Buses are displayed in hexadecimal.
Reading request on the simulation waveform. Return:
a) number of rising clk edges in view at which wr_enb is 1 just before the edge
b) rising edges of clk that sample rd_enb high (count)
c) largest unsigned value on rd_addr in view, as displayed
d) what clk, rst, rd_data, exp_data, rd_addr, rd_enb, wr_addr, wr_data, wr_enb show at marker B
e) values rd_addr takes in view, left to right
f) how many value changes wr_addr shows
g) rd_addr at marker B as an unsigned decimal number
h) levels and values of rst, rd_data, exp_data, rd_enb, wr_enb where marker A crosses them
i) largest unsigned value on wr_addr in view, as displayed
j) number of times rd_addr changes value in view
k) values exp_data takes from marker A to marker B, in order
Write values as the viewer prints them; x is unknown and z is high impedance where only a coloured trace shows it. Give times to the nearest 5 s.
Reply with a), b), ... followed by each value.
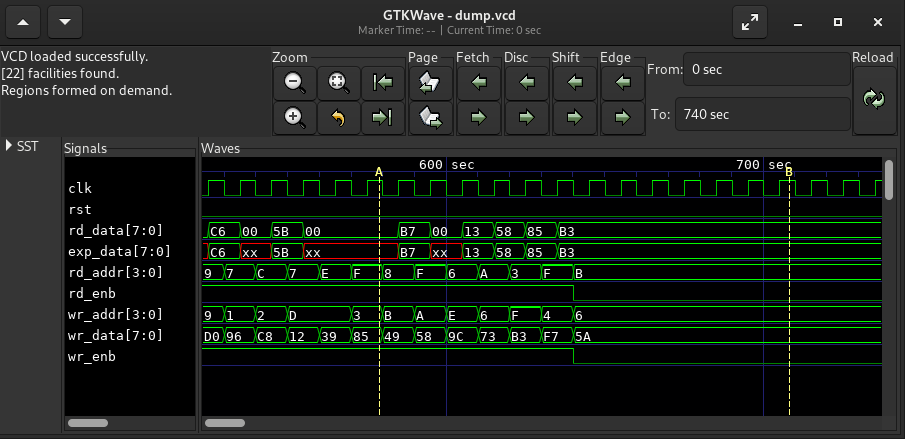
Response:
a) 12
b) 12
c) F
d) clk=1, rst=0, rd_data=B3, exp_data=B3, rd_addr=B, rd_enb=0, wr_addr=6, wr_data=5A, wr_enb=0
e) 9, 7, C, 7, E, F, 8, F, 6, A, 3, F, B
f) 11
g) 11
h) rst=0, rd_data=00, exp_data=xx, rd_enb=1, wr_enb=1
i) F
j) 12
k) xx, B7, xx, 13, 58, 85, B3
